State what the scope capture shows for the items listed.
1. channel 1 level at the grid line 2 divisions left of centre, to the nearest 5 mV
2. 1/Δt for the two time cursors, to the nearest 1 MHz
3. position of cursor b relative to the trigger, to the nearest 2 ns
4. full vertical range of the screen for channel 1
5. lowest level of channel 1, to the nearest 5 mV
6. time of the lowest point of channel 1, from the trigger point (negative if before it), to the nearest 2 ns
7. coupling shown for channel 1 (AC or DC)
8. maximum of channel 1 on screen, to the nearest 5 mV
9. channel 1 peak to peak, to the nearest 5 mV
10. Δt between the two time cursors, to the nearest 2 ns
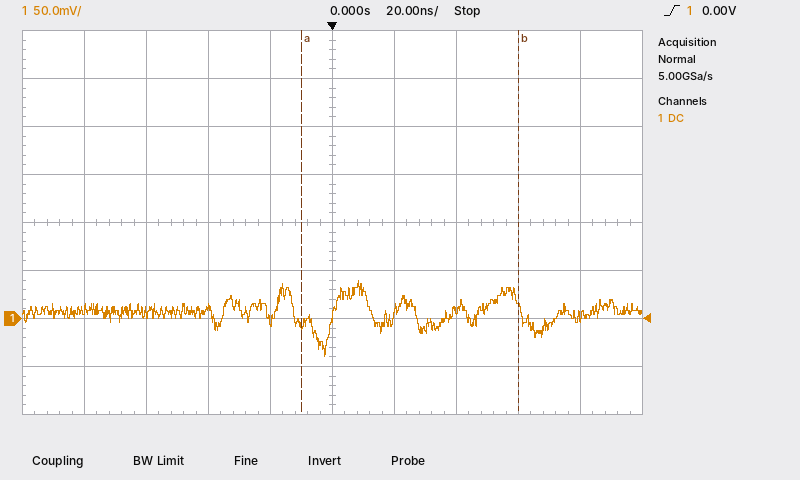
10 mV
14 MHz
+60 ns
400 mV
-40 mV
-2 ns
DC
40 mV
80 mV
70 ns
